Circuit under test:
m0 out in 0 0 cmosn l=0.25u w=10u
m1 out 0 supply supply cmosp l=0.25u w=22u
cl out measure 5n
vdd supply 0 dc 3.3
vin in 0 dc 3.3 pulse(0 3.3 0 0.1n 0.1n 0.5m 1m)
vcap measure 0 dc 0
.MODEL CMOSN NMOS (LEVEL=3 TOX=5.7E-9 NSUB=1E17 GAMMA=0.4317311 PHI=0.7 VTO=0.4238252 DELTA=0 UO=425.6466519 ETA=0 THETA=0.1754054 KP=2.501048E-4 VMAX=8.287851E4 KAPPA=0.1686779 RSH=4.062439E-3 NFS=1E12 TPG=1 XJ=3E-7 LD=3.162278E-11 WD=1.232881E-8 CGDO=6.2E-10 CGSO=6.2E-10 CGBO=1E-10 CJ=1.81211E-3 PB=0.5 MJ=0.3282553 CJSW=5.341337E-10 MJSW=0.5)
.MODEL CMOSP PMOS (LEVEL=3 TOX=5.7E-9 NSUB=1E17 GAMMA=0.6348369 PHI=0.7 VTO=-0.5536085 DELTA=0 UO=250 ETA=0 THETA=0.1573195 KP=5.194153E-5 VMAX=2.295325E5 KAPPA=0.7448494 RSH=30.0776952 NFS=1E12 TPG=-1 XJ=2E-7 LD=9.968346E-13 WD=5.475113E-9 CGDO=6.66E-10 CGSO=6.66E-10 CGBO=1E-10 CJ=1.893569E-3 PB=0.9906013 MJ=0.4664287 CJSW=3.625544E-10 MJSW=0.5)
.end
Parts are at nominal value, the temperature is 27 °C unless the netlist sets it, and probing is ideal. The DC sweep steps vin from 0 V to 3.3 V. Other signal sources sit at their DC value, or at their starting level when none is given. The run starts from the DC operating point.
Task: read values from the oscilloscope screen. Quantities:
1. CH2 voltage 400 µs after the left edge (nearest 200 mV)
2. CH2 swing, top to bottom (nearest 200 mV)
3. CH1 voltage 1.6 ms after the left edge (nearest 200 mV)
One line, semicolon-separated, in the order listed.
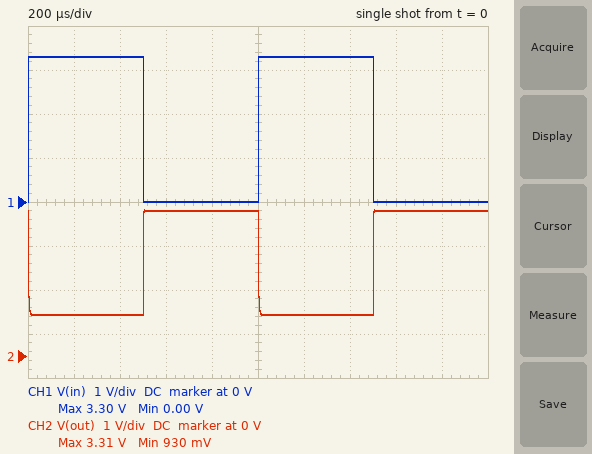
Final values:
1.0 V; 2.4 V; 0 V
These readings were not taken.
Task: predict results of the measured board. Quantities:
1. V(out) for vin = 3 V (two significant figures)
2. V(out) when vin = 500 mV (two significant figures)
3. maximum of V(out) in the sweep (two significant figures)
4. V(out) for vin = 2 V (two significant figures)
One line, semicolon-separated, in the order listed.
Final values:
1.4 V; 3.3 V; 3.3 V; 2.4 V
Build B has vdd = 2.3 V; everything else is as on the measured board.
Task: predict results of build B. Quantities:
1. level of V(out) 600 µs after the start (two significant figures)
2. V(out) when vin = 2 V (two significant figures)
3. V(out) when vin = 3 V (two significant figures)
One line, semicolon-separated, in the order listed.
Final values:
2.3 V; 910 mV; 300 mV
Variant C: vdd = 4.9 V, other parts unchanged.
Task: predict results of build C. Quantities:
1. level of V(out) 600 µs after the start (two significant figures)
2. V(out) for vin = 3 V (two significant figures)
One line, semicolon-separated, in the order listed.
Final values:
4.9 V; 3.5 V
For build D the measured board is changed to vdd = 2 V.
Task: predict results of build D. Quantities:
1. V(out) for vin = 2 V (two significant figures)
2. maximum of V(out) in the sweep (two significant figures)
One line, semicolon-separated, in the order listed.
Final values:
390 mV; 2.0 V
